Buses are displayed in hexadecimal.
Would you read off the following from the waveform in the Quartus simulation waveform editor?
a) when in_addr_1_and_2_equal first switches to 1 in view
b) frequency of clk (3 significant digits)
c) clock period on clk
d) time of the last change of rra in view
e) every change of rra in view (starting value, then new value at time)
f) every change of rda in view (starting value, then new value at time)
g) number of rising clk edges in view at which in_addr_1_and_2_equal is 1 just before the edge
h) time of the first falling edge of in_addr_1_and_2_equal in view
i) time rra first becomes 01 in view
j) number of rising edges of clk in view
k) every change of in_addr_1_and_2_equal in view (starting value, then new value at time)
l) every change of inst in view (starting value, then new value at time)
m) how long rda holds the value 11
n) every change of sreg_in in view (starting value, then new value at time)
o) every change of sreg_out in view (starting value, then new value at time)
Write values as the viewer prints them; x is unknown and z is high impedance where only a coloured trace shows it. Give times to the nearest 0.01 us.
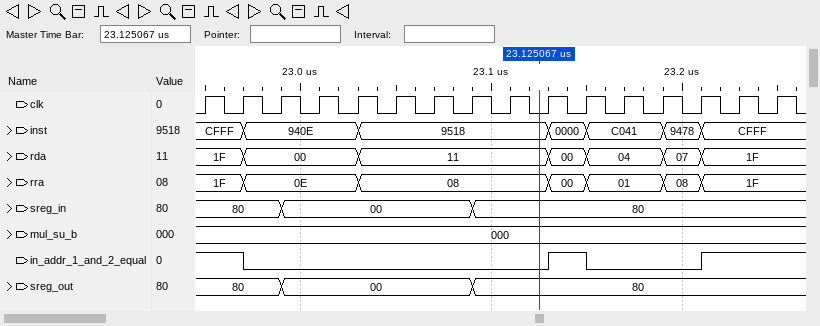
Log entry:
23.13 us
50.0 MHz
0.02 us
23.21 us
1F, 0E at 22.97 us, 08 at 23.03 us, 00 at 23.13 us, 01 at 23.15 us, 08 at 23.19 us, 1F at 23.21 us
1F, 00 at 22.97 us, 11 at 23.03 us, 00 at 23.13 us, 04 at 23.15 us, 07 at 23.19 us, 1F at 23.21 us
5
22.97 us
23.15 us
16
1, 0 at 22.97 us, 1 at 23.13 us, 0 at 23.15 us, 1 at 23.21 us
CFFF, 940E at 22.97 us, 9518 at 23.03 us, 0000 at 23.13 us, C041 at 23.15 us, 9478 at 23.19 us, CFFF at 23.21 us
0.1 us
80, 00 at 22.99 us, 80 at 23.09 us
80, 00 at 22.99 us, 80 at 23.09 us
